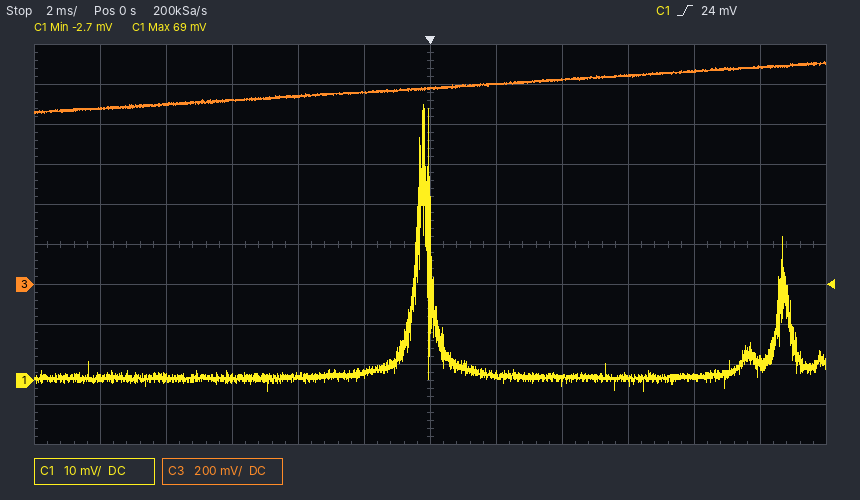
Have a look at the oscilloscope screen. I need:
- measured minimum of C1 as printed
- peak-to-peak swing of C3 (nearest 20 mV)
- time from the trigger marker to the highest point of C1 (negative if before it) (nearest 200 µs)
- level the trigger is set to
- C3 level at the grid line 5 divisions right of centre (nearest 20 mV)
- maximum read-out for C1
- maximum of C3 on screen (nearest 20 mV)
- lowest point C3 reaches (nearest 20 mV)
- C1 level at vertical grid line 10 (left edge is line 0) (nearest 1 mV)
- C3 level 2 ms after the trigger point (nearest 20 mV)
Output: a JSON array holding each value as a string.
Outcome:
["-2.7 mV", "260 mV", "-200 µs", "24 mV", "1.08 V", "69 mV", "1.12 V", "860 mV", "1 mV", "1.00 V"]
